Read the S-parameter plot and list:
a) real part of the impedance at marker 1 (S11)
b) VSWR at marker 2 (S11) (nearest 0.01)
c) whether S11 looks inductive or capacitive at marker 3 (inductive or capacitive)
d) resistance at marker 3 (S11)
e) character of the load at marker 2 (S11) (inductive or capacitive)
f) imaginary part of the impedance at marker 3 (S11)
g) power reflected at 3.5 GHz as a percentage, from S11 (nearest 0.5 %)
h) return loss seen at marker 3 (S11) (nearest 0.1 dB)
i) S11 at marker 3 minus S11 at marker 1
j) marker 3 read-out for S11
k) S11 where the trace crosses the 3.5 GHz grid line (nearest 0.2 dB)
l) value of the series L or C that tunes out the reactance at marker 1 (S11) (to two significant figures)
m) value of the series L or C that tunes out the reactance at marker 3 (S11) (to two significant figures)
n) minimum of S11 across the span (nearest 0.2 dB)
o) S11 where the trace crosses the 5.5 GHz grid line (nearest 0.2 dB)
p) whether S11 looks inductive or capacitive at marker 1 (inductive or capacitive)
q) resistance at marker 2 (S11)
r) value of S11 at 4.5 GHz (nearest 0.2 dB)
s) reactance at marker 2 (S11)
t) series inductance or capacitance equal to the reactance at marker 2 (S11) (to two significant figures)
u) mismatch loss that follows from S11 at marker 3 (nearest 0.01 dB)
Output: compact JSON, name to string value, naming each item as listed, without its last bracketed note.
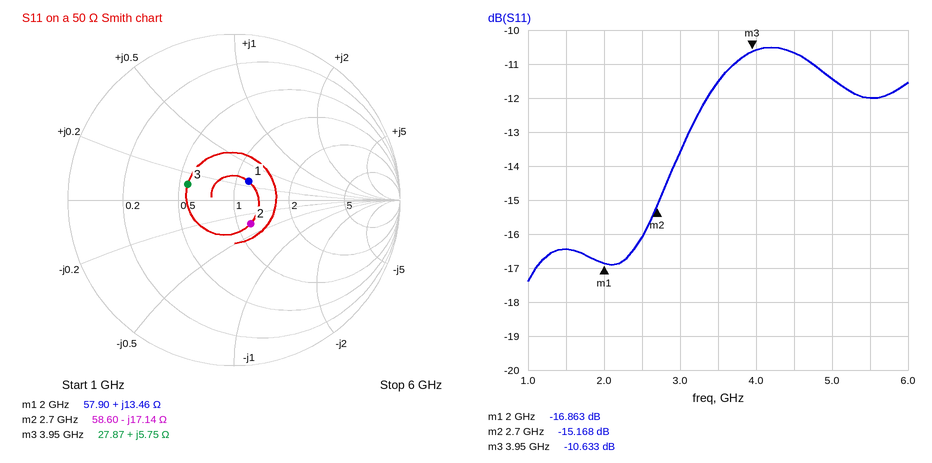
{"real part of the impedance at marker 1": "57.90 Ω", "VSWR at marker 2 (S11)": "1.42", "whether S11 looks inductive or capacitive at marker 3": "inductive", "resistance at marker 3": "27.87 Ω", "character of the load at marker 2 (S11)": "capacitive", "imaginary part of the impedance at marker 3": "+5.75 Ω", "power reflected at 3.5 GHz as a percentage, from S11": "7.0 %", "return loss seen at marker 3 (S11)": "10.7 dB", "S11 at marker 3 minus S11 at marker 1": "6.230 dB", "marker 3 read-out for S11": "-10.633 dB", "S11 where the trace crosses the 3.5 GHz grid line": "-11.6 dB", "value of the series L or C that tunes out the reactance at marker 1 (S11)": "5.9 pF", "value of the series L or C that tunes out the reactance at marker 3 (S11)": "7.0 pF", "minimum of S11 across the span": "-17.4 dB", "S11 where the trace crosses the 5.5 GHz grid line": "-12.0 dB", "whether S11 looks inductive or capacitive at marker 1": "inductive", "resistance at marker 2": "58.60 Ω", "value of S11 at 4.5 GHz": "-10.6 dB", "reactance at marker 2": "-17.14 Ω", "series inductance or capacitance equal to the reactance at marker 2 (S11)": "3.4 pF", "mismatch loss that follows from S11 at marker 3": "0.39 dB"}
